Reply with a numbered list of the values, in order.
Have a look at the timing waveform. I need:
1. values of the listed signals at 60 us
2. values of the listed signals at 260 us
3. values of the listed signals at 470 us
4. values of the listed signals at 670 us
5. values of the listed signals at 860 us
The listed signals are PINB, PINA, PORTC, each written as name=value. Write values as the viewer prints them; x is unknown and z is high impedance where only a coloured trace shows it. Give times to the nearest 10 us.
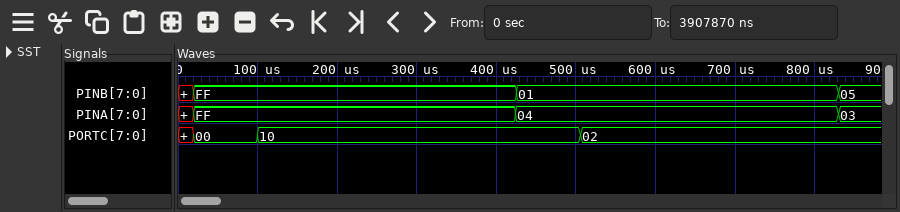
1. PINB=FF, PINA=FF, PORTC=00
2. PINB=FF, PINA=FF, PORTC=10
3. PINB=01, PINA=04, PORTC=10
4. PINB=01, PINA=04, PORTC=02
5. PINB=05, PINA=03, PORTC=02
